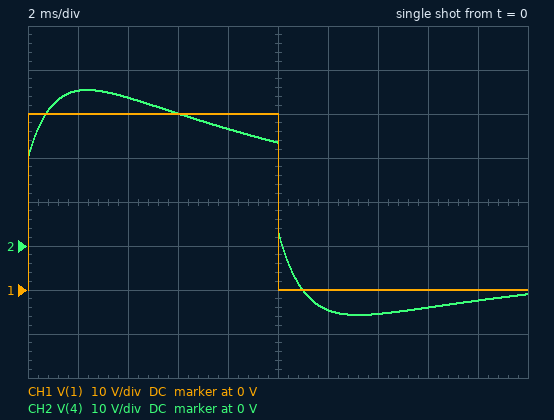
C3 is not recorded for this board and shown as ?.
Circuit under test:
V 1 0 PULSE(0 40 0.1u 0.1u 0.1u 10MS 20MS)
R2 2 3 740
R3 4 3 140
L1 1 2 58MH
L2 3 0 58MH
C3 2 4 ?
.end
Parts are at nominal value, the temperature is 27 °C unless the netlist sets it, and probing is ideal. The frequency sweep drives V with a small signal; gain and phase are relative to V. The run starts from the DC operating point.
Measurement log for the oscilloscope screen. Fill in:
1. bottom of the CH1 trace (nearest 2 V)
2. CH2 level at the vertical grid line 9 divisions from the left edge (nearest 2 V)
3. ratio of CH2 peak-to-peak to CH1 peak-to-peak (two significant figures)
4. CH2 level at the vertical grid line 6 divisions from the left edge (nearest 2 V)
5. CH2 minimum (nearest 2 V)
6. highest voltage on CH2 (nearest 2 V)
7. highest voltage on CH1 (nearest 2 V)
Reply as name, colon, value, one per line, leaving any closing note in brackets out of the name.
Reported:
bottom of the CH1 trace: 0 V
CH2 level at the vertical grid line 9 divisions from the left edge: -12 V
ratio of CH2 peak-to-peak to CH1 peak-to-peak: 1.3
CH2 level at the vertical grid line 6 divisions from the left edge: -14 V
CH2 minimum: -16 V
highest voltage on CH2: 36 V
highest voltage on CH1: 40 V
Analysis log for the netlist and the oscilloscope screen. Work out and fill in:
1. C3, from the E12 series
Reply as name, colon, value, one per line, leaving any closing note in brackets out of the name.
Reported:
C3, from the E12 series: 120 µF
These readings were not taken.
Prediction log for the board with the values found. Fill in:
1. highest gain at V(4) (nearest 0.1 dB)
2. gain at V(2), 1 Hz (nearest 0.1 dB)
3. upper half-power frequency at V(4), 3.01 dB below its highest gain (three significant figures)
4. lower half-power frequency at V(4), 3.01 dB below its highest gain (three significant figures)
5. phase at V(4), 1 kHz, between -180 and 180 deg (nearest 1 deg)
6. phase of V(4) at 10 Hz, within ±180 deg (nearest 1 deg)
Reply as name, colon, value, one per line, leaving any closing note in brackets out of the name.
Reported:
highest gain at V(4): 0 dB
gain at V(2), 1 Hz: 0 dB
upper half-power frequency at V(4), 3.01 dB below its highest gain: 239 Hz
lower half-power frequency at V(4), 3.01 dB below its highest gain: 9.02 Hz
phase at V(4), 1 kHz, between -180 and 180 deg: -9 deg
phase of V(4) at 10 Hz, within ±180 deg: 43 deg
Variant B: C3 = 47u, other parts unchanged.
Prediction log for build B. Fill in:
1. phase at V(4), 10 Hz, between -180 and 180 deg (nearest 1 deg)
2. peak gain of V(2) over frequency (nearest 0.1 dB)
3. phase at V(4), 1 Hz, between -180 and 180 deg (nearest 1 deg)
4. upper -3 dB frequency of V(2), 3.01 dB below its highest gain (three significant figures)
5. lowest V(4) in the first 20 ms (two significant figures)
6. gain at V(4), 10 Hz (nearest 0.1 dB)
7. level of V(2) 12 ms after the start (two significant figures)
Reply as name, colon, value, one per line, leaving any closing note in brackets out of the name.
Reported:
phase at V(4), 10 Hz, between -180 and 180 deg: 68 deg
peak gain of V(2) over frequency: 0.3 dB
phase at V(4), 1 Hz, between -180 and 180 deg: 88 deg
upper -3 dB frequency of V(2), 3.01 dB below its highest gain: 209 Hz
lowest V(4) in the first 20 ms: -26 V
gain at V(4), 10 Hz: -8.1 dB
level of V(2) 12 ms after the start: 1.7 V
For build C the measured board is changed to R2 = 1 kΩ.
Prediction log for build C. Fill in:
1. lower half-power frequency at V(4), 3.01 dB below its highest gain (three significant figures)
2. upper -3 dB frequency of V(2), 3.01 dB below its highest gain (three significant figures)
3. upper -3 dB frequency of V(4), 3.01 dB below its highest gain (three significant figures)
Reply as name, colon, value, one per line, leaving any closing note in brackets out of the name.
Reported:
lower half-power frequency at V(4), 3.01 dB below its highest gain: 9.05 Hz
upper -3 dB frequency of V(2), 3.01 dB below its highest gain: 227 Hz
upper -3 dB frequency of V(4), 3.01 dB below its highest gain: 248 Hz
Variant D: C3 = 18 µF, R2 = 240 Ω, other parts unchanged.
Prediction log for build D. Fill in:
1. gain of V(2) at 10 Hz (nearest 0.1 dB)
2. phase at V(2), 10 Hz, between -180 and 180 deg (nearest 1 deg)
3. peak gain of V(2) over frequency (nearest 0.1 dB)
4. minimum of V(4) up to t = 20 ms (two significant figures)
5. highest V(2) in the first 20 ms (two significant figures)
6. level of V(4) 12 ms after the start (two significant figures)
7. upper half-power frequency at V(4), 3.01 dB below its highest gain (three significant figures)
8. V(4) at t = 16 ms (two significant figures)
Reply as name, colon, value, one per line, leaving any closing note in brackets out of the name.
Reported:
gain of V(2) at 10 Hz: 0 dB
phase at V(2), 10 Hz, between -180 and 180 deg: -1 deg
peak gain of V(2) over frequency: 0.3 dB
minimum of V(4) up to t = 20 ms: -28 V
highest V(2) in the first 20 ms: 42 V
level of V(4) 12 ms after the start: -25 V
upper half-power frequency at V(4), 3.01 dB below its highest gain: 257 Hz
V(4) at t = 16 ms: -4.6 V
